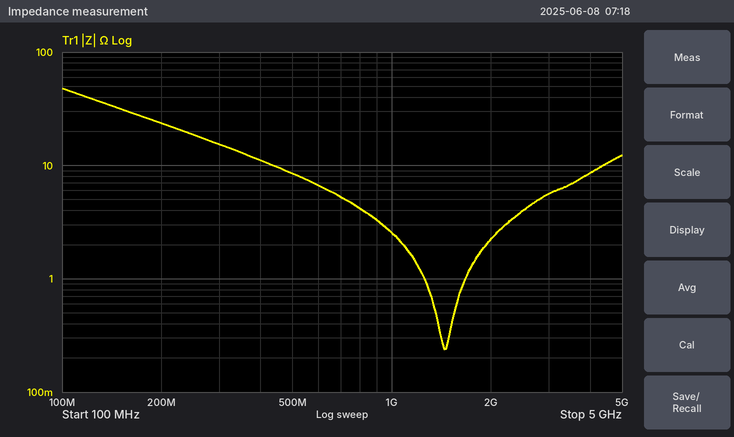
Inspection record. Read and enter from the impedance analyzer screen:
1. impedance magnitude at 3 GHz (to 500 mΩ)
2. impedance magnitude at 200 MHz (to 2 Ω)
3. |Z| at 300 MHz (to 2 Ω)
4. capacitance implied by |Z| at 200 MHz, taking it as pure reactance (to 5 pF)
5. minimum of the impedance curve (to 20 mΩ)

5.5 Ω
24 Ω
16 Ω
35 pF
240 mΩ
